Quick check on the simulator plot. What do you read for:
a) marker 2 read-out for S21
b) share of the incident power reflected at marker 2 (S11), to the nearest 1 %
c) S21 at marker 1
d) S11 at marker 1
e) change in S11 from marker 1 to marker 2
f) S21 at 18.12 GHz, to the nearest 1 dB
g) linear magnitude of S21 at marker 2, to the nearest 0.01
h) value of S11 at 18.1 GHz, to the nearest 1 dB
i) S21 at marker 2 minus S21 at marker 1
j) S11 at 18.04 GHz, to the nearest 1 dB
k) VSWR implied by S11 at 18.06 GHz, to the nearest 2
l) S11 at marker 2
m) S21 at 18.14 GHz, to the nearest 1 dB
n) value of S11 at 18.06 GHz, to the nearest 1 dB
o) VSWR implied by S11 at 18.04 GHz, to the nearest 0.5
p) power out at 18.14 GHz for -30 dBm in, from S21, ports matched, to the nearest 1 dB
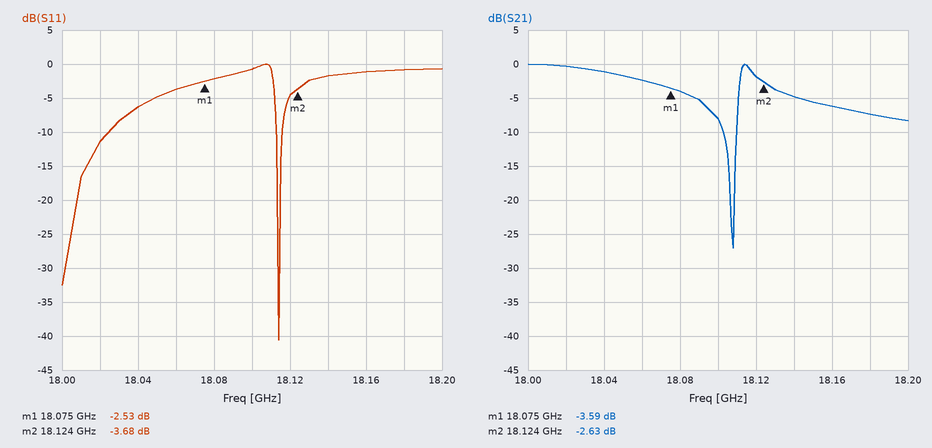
-2.63 dB
43 %
-3.59 dB
-2.53 dB
-1.15 dB
-2 dB
0.74
-1 dB
0.96 dB
-6 dB
4
-3.68 dB
-5 dB
-4 dB
3.0
-35 dBm
